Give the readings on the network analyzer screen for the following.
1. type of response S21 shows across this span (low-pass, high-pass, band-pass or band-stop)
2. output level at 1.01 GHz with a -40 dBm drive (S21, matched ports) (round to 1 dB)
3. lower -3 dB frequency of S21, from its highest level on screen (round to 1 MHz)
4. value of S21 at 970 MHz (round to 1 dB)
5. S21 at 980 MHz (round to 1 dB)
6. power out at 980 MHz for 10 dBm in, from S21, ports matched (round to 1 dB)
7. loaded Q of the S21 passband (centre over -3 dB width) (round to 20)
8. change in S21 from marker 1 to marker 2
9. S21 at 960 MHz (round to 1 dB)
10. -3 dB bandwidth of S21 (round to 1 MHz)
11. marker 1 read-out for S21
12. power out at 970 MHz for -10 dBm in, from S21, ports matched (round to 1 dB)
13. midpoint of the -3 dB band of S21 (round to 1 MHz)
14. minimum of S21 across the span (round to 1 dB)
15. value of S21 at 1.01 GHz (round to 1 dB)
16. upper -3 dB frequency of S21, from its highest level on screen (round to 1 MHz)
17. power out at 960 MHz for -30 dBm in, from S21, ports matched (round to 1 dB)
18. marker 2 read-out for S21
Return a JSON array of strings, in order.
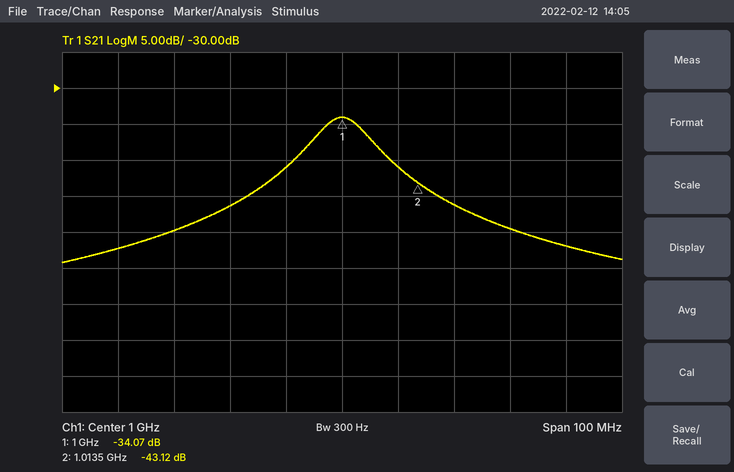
["band-pass", "-81 dBm", "995 MHz", "-50 dB", "-46 dB", "-36 dBm", "100", "-9.05 dB", "-52 dB", "10 MHz", "-34.07 dB", "-60 dBm", "1.000 GHz", "-54 dB", "-41 dB", "1.005 GHz", "-82 dBm", "-43.12 dB"]
